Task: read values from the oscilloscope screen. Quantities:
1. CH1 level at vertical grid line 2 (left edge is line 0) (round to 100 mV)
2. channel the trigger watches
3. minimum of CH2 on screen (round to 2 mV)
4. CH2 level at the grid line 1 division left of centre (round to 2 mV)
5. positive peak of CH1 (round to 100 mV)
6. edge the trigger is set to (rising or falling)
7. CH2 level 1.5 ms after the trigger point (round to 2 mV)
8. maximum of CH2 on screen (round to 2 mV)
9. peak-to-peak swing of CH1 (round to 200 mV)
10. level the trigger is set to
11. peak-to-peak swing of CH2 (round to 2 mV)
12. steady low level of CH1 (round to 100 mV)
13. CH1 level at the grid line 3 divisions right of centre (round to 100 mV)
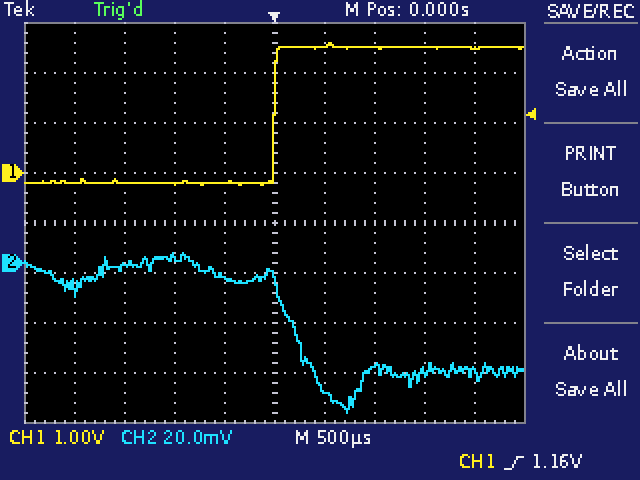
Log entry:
-200 mV
CH1
-60 mV
-6 mV
2.6 V
rising
-44 mV
4 mV
2.8 V
1.16 V
64 mV
-200 mV
2.5 V
